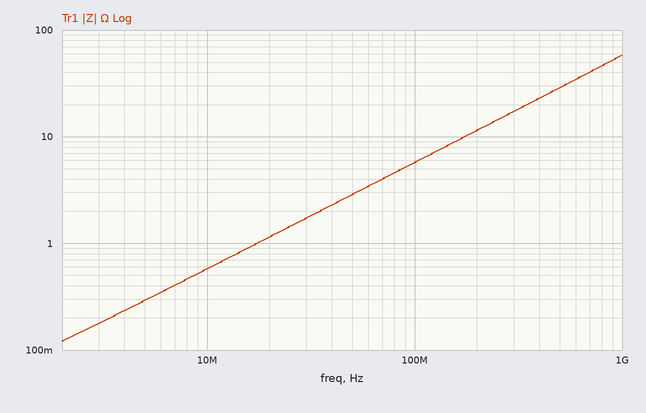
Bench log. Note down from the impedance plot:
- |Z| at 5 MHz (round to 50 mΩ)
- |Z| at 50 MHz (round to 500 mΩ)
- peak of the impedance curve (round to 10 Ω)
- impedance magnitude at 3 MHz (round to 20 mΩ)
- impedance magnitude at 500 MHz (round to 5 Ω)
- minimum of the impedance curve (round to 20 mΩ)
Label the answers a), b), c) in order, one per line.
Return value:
a) 300 mΩ
b) 3.0 Ω
c) 60 Ω
d) 180 mΩ
e) 30 Ω
f) 120 mΩ
